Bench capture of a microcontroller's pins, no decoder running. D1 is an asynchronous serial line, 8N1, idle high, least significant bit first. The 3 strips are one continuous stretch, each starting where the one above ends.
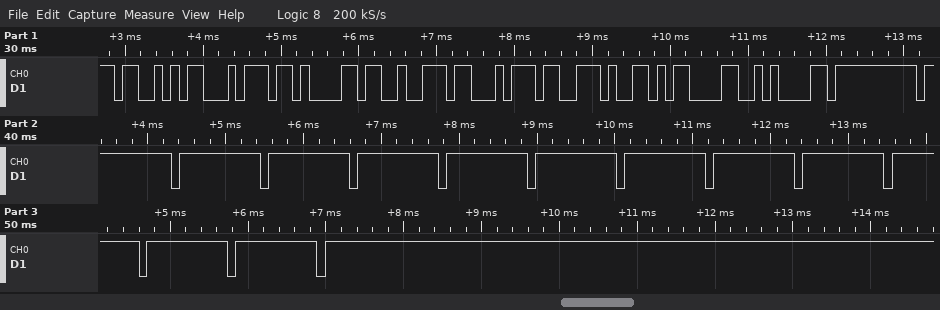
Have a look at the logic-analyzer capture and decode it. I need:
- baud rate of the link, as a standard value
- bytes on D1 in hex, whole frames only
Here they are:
9600 baud
0x53 0x74 0x61 0x72 0x74 0x2E 0x0D 0x0A 0xFF 0xFF 0xFF 0xFF 0xFF 0xFF 0xFF 0xFF 0xFF 0xFF 0xFF 0xFF 0xFF 0xFF
